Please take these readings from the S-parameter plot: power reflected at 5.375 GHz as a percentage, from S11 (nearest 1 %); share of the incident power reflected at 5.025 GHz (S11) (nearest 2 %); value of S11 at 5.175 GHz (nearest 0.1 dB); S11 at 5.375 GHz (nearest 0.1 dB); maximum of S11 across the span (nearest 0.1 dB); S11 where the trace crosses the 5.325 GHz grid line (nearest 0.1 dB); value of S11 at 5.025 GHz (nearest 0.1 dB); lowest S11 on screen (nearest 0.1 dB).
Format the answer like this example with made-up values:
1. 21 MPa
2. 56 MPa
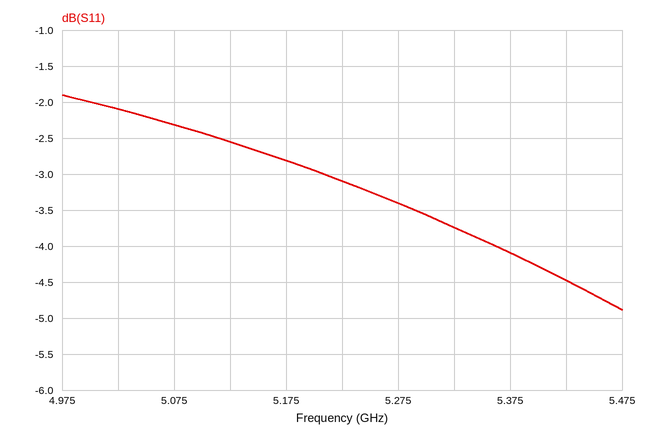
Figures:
1. 39 %
2. 62 %
3. -2.8 dB
4. -4.1 dB
5. -1.9 dB
6. -3.7 dB
7. -2.1 dB
8. -4.9 dB
